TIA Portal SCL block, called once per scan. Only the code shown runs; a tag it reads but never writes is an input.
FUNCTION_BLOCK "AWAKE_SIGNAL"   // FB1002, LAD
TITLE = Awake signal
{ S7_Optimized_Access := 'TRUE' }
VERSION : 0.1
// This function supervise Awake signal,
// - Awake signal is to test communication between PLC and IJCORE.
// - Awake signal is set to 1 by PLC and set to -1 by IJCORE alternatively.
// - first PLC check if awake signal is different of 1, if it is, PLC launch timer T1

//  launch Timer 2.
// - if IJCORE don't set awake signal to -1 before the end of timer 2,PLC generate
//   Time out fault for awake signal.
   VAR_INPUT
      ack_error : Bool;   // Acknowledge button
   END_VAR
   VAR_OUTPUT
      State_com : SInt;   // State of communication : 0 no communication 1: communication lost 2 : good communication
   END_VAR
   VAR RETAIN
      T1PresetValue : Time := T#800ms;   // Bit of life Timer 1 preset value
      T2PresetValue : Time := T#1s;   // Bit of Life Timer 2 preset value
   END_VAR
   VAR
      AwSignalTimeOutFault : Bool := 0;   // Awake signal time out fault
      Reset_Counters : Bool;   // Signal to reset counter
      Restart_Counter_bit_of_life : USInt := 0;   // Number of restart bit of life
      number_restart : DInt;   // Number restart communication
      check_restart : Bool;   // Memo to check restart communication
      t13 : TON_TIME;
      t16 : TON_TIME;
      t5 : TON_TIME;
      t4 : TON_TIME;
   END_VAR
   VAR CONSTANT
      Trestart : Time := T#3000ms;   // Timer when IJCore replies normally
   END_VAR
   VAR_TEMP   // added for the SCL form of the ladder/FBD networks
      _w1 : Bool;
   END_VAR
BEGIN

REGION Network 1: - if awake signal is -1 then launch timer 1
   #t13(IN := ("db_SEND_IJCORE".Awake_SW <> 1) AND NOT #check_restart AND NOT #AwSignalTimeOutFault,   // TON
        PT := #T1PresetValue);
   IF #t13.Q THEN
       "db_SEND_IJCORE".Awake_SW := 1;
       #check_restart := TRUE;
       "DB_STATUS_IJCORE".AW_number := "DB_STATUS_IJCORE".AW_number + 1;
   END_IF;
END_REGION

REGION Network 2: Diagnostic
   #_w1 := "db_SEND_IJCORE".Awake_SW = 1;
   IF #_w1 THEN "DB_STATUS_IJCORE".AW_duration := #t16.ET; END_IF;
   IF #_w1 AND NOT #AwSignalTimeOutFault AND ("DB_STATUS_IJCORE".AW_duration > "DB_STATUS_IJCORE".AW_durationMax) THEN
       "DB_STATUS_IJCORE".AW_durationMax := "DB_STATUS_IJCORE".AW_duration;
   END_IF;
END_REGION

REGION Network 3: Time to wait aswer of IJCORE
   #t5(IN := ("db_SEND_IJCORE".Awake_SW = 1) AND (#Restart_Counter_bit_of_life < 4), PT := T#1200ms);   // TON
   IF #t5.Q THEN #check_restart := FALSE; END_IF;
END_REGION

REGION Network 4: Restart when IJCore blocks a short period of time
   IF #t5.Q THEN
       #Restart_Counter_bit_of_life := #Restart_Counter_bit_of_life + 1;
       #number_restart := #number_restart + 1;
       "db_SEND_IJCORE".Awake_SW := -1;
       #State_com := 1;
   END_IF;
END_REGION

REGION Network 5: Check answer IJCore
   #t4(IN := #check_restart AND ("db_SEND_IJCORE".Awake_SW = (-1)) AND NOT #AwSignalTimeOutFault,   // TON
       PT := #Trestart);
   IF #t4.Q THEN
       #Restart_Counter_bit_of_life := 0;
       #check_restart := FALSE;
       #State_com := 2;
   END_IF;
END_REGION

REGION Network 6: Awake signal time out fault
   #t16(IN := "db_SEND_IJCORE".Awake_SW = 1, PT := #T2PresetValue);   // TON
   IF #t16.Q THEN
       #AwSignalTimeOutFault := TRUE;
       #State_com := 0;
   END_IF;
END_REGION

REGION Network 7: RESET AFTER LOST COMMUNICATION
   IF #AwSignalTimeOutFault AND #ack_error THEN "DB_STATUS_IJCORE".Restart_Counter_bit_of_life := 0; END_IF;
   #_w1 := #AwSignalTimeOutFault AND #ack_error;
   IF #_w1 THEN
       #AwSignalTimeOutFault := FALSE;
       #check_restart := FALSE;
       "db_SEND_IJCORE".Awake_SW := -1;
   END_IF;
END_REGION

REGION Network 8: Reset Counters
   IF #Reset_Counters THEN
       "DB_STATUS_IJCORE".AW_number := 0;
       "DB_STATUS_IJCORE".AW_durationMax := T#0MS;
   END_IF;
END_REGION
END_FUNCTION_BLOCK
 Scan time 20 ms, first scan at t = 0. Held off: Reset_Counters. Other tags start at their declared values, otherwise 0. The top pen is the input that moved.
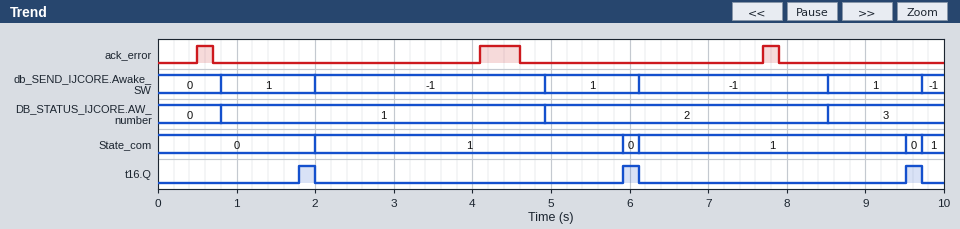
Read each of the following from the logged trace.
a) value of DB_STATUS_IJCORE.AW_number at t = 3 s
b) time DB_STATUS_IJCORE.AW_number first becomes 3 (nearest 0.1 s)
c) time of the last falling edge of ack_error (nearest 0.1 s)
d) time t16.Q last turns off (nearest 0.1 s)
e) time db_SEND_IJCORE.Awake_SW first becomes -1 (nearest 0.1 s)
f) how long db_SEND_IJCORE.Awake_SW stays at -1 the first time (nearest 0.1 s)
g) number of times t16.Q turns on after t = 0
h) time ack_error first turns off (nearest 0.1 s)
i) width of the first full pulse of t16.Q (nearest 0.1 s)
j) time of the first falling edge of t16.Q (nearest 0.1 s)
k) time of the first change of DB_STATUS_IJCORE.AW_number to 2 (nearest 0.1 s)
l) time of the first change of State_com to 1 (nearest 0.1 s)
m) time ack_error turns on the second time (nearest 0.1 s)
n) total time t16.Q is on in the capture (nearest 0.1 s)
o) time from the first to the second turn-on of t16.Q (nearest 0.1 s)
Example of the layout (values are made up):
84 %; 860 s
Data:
1; 8.5 s; 7.9 s; 9.7 s; 2.0 s; 2.9 s; 3; 0.7 s; 0.2 s; 2.0 s; 4.9 s; 2.0 s; 4.1 s; 0.6 s; 4.1 s
